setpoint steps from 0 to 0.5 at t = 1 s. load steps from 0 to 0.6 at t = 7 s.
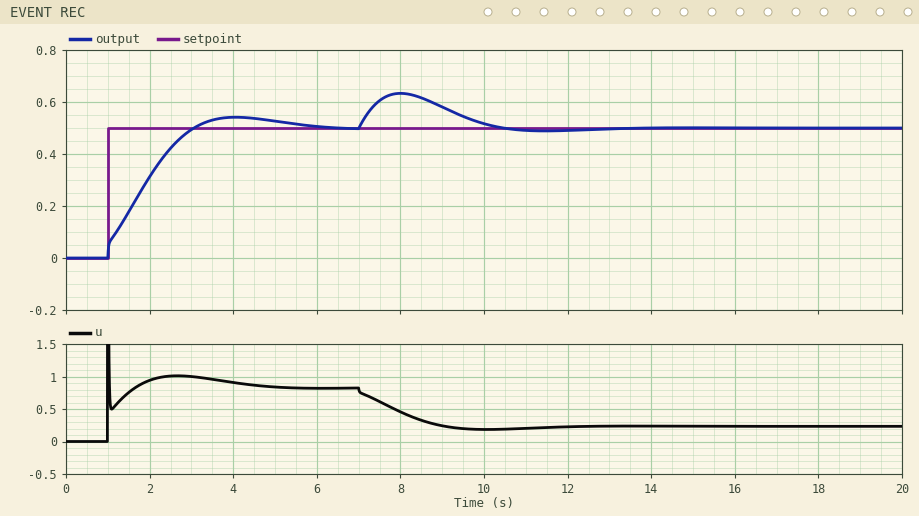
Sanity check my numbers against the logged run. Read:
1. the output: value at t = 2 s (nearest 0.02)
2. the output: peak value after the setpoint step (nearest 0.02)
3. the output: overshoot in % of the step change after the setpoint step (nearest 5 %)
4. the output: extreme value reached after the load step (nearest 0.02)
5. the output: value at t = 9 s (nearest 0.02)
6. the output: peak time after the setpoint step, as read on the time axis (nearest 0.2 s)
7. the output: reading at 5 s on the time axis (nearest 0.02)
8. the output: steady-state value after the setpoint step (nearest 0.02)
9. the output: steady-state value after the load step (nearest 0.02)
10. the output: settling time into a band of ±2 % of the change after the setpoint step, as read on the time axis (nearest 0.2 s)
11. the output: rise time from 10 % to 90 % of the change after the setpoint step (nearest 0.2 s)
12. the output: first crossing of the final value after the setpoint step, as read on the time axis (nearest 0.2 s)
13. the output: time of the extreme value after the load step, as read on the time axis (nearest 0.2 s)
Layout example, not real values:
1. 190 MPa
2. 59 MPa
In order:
1. 0.32
2. 0.54
3. 10 %
4. 0.64
5. 0.58
6. 4.0 s
7. 0.52
8. 0.50
9. 0.50
10. 5.8 s
11. 1.6 s
12. 3.0 s
13. 8.0 s
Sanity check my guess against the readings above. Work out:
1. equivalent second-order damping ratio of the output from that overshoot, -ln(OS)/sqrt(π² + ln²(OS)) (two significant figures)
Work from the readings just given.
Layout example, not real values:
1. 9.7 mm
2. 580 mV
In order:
1. 0.59
